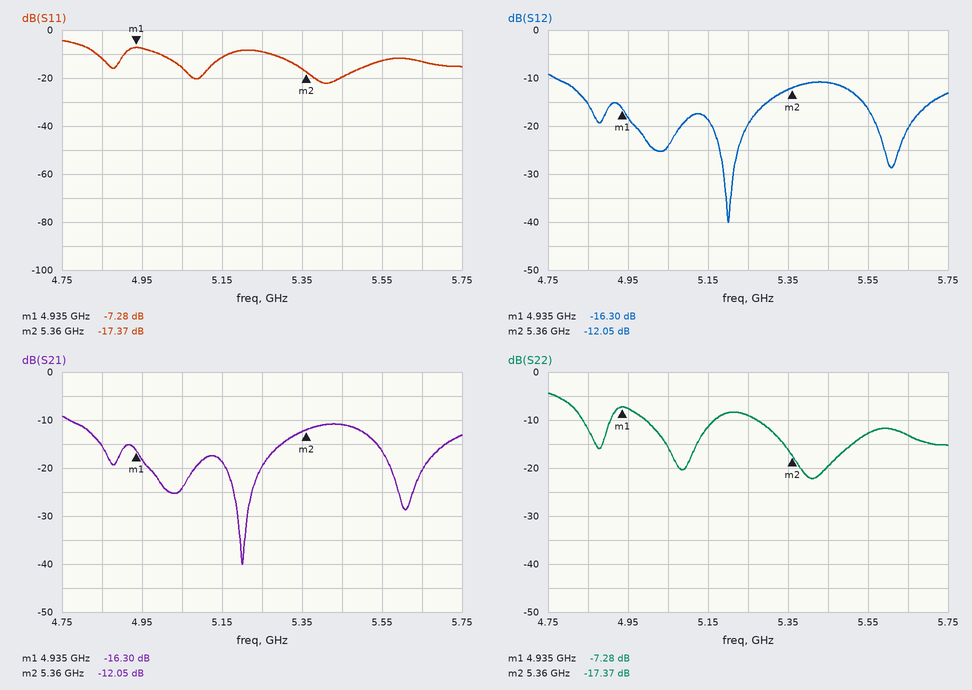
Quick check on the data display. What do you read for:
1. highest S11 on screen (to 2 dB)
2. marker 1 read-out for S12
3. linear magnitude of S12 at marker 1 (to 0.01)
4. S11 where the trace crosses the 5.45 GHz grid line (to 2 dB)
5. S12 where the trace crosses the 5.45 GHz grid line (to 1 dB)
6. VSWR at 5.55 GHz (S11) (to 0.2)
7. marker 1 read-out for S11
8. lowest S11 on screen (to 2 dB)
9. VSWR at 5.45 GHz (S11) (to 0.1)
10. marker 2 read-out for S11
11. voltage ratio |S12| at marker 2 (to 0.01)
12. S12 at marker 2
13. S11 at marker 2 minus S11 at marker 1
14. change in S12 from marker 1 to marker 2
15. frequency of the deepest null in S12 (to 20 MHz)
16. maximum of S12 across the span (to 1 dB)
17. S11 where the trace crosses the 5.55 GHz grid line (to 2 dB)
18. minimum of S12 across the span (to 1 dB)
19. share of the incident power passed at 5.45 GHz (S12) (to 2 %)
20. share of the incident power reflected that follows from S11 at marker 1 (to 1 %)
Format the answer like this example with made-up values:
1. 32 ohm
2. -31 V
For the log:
1. -4 dB
2. -16.30 dB
3. 0.15
4. -20 dB
5. -11 dB
6. 1.6
7. -7.28 dB
8. -22 dB
9. 1.2
10. -17.37 dB
11. 0.25
12. -12.05 dB
13. -10.09 dB
14. 4.25 dB
15. 5.20 GHz
16. -9 dB
17. -12 dB
18. -40 dB
19. 8 %
20. 19 %
